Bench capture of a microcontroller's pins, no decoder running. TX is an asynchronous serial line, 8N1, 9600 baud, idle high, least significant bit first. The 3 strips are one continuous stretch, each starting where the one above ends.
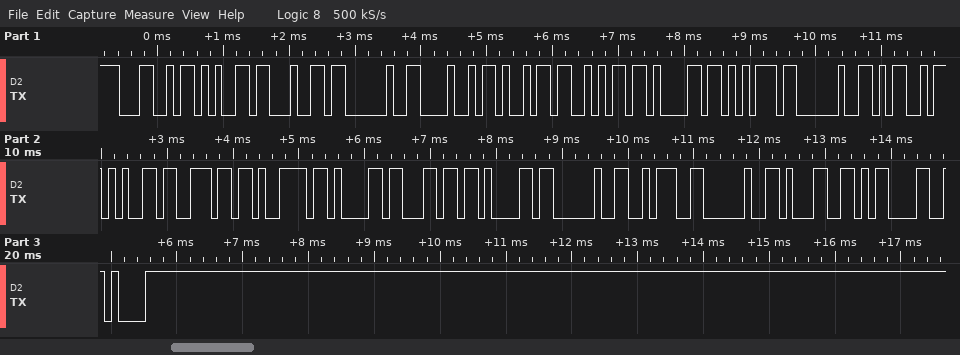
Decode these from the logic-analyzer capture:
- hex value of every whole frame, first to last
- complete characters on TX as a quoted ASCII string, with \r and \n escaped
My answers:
4C 65 64 20 48 69 6A 61 75 20 4D 65 6E 79 61 6C 61 20 3A 20 31 0D 0A
"Led Hijau Menyala : 1\r\n"
